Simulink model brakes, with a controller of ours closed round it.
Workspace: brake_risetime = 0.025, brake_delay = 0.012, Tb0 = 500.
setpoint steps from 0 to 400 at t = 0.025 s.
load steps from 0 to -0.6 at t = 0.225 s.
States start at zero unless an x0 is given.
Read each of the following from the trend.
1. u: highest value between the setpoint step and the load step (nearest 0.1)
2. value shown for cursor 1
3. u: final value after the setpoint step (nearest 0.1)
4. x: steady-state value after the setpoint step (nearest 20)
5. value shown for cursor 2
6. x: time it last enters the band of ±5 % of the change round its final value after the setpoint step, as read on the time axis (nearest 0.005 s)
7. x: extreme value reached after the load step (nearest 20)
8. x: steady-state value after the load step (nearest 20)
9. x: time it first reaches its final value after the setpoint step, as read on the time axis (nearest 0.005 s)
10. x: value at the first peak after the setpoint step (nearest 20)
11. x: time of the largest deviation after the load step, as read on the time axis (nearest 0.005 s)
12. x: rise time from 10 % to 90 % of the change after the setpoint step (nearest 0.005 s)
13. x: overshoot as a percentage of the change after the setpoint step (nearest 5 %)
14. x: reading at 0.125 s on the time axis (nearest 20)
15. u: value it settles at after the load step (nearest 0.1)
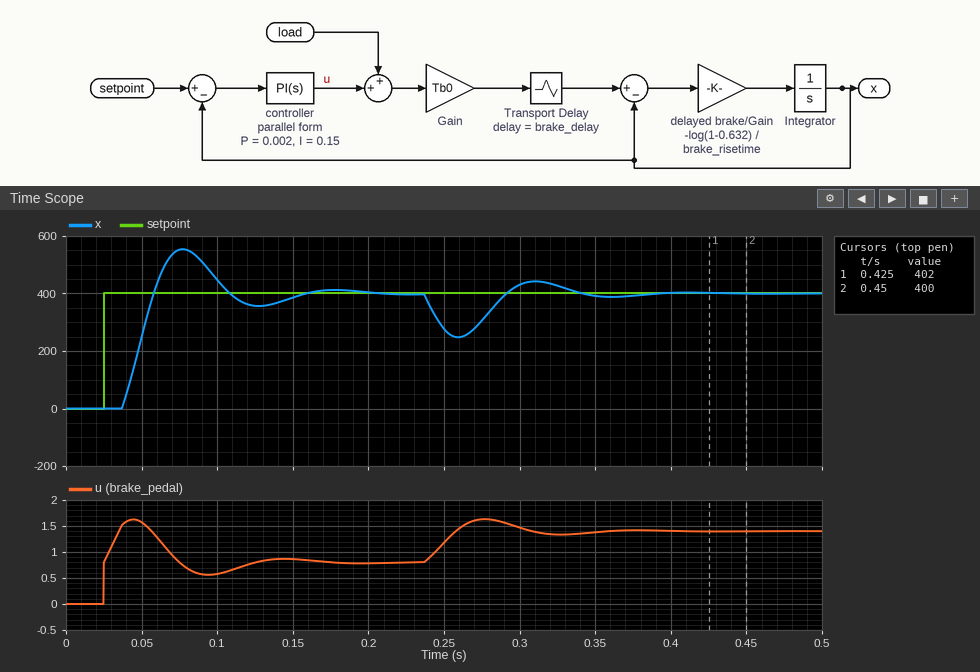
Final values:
1.6
402
0.8
400
400
0.145 s
240
400
0.060 s
560
0.260 s
0.015 s
40 %
360
1.4
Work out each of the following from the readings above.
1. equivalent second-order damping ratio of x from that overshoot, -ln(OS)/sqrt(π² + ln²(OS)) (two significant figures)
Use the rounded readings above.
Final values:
0.28
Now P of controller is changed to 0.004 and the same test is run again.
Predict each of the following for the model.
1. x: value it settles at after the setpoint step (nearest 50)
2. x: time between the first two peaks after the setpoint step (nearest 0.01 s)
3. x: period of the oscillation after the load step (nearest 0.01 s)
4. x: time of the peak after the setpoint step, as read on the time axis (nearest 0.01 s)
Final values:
400
0.06 s
0.06 s
0.06 s
